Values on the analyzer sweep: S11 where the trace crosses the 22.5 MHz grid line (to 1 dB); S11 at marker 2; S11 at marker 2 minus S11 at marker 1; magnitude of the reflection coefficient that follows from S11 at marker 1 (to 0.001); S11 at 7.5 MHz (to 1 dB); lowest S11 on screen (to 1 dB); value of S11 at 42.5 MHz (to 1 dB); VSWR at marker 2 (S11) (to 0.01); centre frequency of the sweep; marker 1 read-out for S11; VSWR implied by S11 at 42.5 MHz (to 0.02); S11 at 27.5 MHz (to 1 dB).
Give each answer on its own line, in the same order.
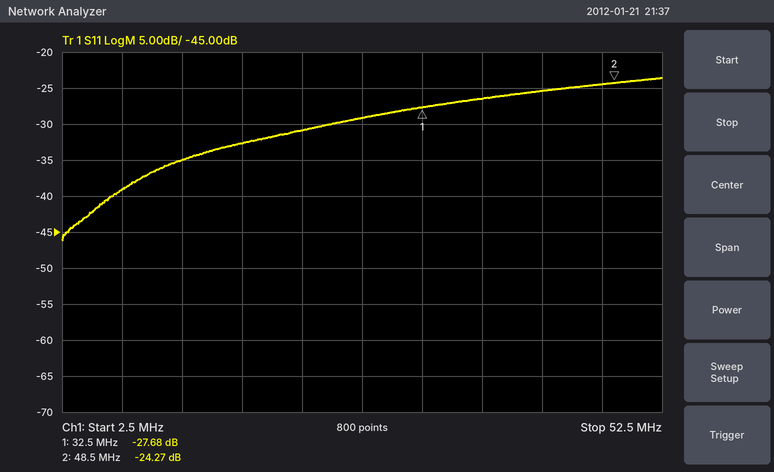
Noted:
-31 dB
-24.27 dB
3.41 dB
0.041
-39 dB
-46 dB
-25 dB
1.13
27.5 MHz
-27.68 dB
1.12
-29 dB
